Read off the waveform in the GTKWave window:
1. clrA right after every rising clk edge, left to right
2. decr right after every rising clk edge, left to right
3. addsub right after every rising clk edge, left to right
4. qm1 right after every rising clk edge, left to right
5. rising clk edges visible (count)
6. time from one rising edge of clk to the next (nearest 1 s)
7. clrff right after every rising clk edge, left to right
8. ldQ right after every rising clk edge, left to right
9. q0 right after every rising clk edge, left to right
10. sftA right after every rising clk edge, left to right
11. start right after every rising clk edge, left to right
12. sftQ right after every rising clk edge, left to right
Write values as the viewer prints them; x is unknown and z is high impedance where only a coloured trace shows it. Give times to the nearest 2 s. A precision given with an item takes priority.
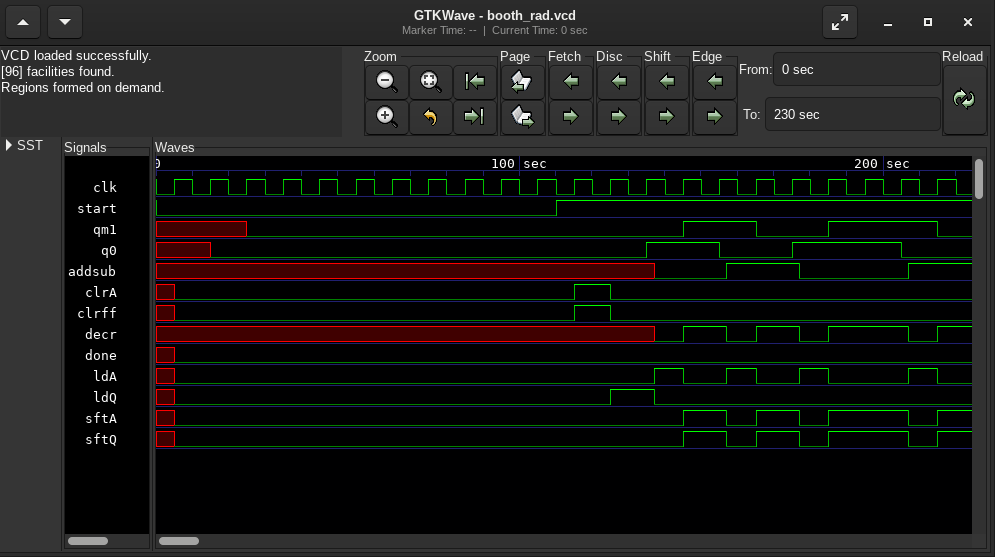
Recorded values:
0 0 0 0 0 0 0 0 0 0 0 1 0 0 0 0 0 0 0 0 0 0
x x x x x x x x x x x x x x 1 1 1 1 1 1 1 1
x x x x x x x x x x x x x x 0 0 1 1 0 0 0 1
x x 0 0 0 0 0 0 0 0 0 0 0 0 1 1 0 0 1 1 1 0
22
10 s
0 0 0 0 0 0 0 0 0 0 0 1 0 0 0 0 0 0 0 0 0 0
0 0 0 0 0 0 0 0 0 0 0 0 1 1 0 0 0 0 0 0 0 0
x 0 0 0 0 0 0 0 0 0 0 0 0 1 1 0 0 1 1 1 0 0
0 0 0 0 0 0 0 0 0 0 0 0 0 0 1 1 1 1 1 1 1 1
0 0 0 0 0 0 0 0 0 0 0 1 1 1 1 1 1 1 1 1 1 1
0 0 0 0 0 0 0 0 0 0 0 0 0 0 1 1 1 1 1 1 1 1
